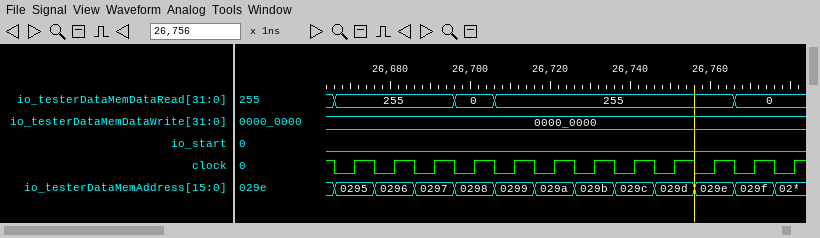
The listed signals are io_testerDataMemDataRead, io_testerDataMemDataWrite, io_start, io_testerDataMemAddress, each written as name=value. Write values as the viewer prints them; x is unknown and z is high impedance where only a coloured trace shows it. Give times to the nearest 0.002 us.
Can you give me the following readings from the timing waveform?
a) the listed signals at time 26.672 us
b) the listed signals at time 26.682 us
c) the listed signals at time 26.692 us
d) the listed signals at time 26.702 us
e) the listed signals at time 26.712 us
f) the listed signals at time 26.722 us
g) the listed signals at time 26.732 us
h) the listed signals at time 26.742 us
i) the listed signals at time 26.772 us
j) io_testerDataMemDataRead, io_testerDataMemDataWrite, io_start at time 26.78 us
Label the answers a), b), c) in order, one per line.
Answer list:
a) io_testerDataMemDataRead=255, io_testerDataMemDataWrite=0000_0000, io_start=0, io_testerDataMemAddress=0295
b) io_testerDataMemDataRead=255, io_testerDataMemDataWrite=0000_0000, io_start=0, io_testerDataMemAddress=0296
c) io_testerDataMemDataRead=255, io_testerDataMemDataWrite=0000_0000, io_start=0, io_testerDataMemAddress=0297
d) io_testerDataMemDataRead=0, io_testerDataMemDataWrite=0000_0000, io_start=0, io_testerDataMemAddress=0298
e) io_testerDataMemDataRead=255, io_testerDataMemDataWrite=0000_0000, io_start=0, io_testerDataMemAddress=0299
f) io_testerDataMemDataRead=255, io_testerDataMemDataWrite=0000_0000, io_start=0, io_testerDataMemAddress=029a
g) io_testerDataMemDataRead=255, io_testerDataMemDataWrite=0000_0000, io_start=0, io_testerDataMemAddress=029b
h) io_testerDataMemDataRead=255, io_testerDataMemDataWrite=0000_0000, io_start=0, io_testerDataMemAddress=029c
i) io_testerDataMemDataRead=0, io_testerDataMemDataWrite=0000_0000, io_start=0, io_testerDataMemAddress=029f
j) io_testerDataMemDataRead=0, io_testerDataMemDataWrite=0000_0000, io_start=0
